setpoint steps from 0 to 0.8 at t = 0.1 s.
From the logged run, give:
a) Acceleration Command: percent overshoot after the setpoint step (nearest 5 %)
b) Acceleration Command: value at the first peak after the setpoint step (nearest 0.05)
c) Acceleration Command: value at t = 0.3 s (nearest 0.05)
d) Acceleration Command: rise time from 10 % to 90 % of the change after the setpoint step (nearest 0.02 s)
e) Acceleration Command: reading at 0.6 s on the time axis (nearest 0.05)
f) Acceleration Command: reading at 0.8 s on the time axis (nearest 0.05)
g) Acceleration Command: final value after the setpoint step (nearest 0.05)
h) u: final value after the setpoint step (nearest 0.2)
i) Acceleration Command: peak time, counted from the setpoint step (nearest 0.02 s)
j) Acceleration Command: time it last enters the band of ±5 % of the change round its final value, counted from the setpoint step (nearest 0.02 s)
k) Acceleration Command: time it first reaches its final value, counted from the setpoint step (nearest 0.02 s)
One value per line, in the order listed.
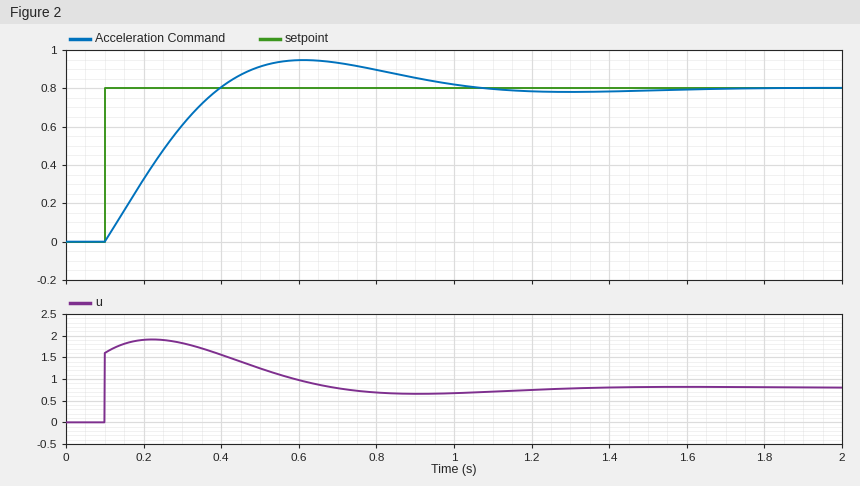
20 %
0.95
0.60
0.22 s
0.95
0.90
0.80
0.8
0.52 s
0.84 s
0.30 s
